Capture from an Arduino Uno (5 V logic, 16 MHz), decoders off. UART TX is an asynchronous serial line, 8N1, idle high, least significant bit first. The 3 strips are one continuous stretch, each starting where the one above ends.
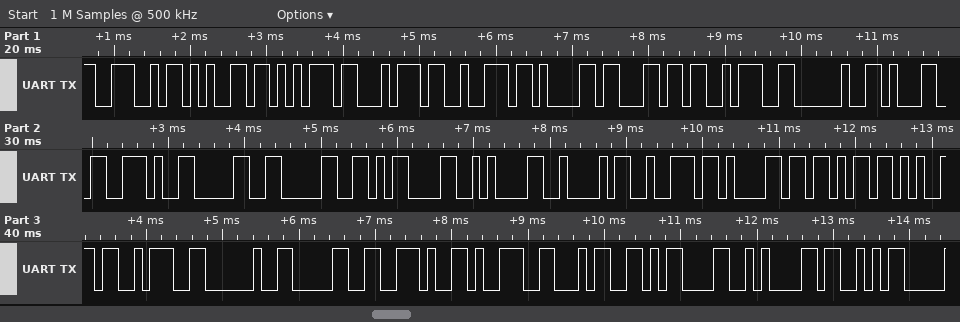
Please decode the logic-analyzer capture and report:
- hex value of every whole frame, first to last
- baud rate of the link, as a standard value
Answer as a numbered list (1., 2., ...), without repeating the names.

1. 4E 65 75 74 72 61 6C 3A 20 31 2E 30 30 0D 0A 42 72 61 6B 65 3A 20 30 2E 39 34 0D 0A 53
2. 9600 baud
